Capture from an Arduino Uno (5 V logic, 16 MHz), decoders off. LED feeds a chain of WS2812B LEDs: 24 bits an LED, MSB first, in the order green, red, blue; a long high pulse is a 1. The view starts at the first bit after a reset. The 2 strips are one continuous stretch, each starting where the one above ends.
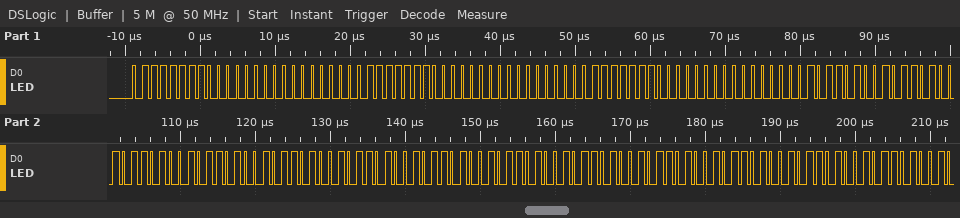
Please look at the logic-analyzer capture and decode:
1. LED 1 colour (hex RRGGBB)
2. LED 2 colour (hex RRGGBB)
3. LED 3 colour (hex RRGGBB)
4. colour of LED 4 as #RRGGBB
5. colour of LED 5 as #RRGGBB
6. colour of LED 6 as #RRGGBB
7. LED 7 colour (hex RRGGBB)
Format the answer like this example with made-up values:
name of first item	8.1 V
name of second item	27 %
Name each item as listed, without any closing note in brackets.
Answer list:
LED 1 colour	#007F00
LED 2 colour	#007F00
LED 3 colour	#007F00
colour of LED 4 as #RRGGBB	#B4B4B4
colour of LED 5 as #RRGGBB	#B4B4B4
colour of LED 6 as #RRGGBB	#B4B4B4
LED 7 colour	#B4B4B4
